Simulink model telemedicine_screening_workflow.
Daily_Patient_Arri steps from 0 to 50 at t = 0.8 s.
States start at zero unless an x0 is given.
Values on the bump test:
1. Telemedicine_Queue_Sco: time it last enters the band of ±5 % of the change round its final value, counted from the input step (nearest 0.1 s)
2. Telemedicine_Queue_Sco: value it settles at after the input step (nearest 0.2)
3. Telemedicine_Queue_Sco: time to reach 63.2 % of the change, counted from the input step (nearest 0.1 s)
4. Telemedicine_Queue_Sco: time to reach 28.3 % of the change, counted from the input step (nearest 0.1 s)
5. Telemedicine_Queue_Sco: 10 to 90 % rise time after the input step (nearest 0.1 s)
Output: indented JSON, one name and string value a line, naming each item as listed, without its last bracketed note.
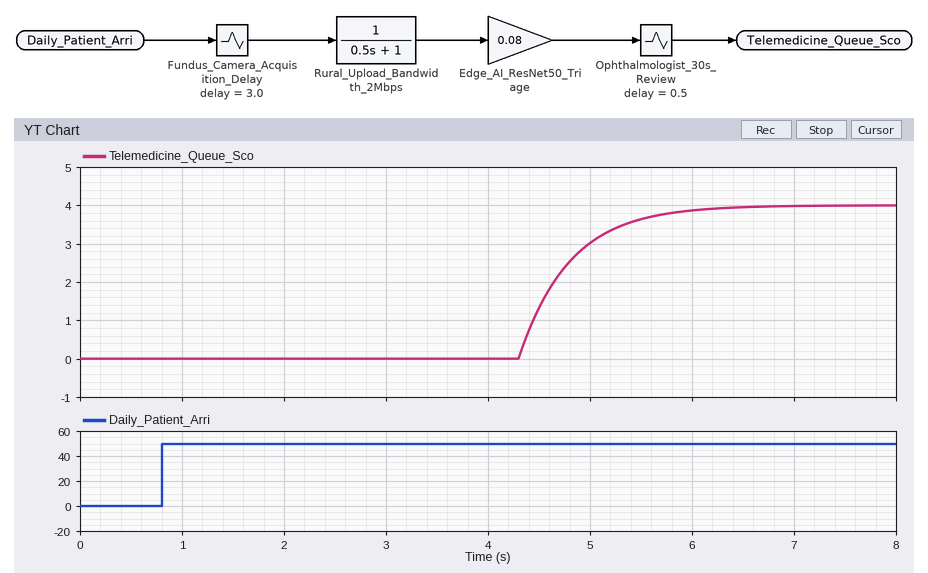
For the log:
{
  "Telemedicine_Queue_Sco: time it last enters the band of ±5 % of the change round its final value, counted from the input step": "5.0 s",
  "Telemedicine_Queue_Sco: value it settles at after the input step": "4.0",
  "Telemedicine_Queue_Sco: time to reach 63.2 % of the change, counted from the input step": "4.0 s",
  "Telemedicine_Queue_Sco: time to reach 28.3 % of the change, counted from the input step": "3.7 s",
  "Telemedicine_Queue_Sco: 10 to 90 % rise time after the input step": "1.1 s"
}
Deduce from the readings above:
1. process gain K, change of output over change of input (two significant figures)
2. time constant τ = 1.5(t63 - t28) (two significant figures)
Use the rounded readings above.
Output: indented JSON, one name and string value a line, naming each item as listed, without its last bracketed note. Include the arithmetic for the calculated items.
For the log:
{
  "process gain K, change of output over change of input": "(4 - 0) / 50 = 0.080",
  "time constant τ = 1.5(t63 - t28)": "1.5 × (4 - 3.7) = 0.45 s"
}
